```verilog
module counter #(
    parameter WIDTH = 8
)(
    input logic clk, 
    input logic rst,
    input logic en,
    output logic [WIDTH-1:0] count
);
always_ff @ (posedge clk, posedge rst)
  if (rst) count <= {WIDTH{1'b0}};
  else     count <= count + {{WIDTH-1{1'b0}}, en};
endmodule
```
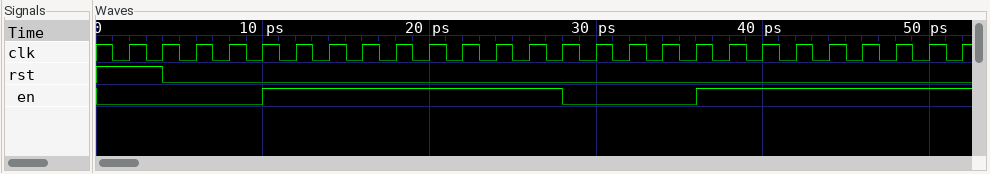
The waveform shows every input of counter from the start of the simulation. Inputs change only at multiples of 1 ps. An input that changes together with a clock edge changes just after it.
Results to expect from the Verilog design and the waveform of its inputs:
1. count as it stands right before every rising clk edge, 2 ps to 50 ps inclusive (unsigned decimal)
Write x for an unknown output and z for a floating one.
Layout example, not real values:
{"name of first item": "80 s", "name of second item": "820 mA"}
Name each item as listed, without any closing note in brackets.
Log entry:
{"count as it stands right before every rising clk edge, 2 ps to 50 ps inclusive": "0, 0, 0, 0, 0, 0, 1, 2, 3, 4, 5, 6, 7, 8, 9, 9, 9, 9, 9, 10, 11, 12, 13, 14, 15"}
